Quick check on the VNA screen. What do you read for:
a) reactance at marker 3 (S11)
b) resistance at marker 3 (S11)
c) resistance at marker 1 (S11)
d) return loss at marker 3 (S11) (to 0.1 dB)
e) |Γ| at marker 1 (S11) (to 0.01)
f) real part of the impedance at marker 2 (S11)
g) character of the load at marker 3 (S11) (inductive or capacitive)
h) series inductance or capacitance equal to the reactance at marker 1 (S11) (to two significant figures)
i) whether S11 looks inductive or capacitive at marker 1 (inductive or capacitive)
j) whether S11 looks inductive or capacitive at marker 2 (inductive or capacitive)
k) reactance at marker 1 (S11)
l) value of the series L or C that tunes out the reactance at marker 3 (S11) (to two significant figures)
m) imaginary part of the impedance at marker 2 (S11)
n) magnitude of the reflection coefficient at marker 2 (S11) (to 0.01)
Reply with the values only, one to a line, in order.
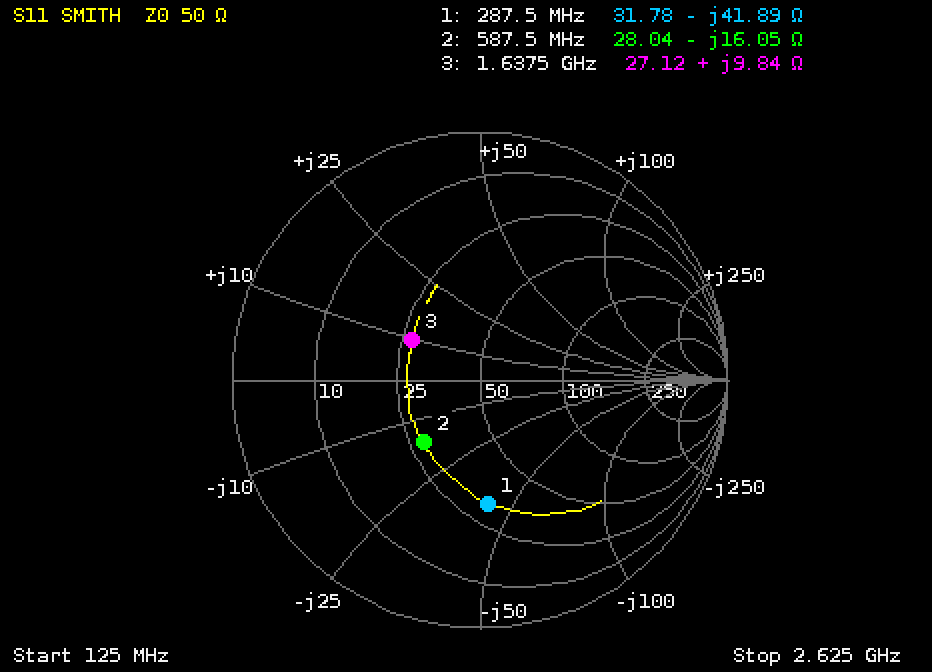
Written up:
+9.84 Ω
27.12 Ω
31.78 Ω
9.9 dB
0.50
28.04 Ω
inductive
13 pF
capacitive
capacitive
-41.89 Ω
9.9 pF
-16.05 Ω
0.34
